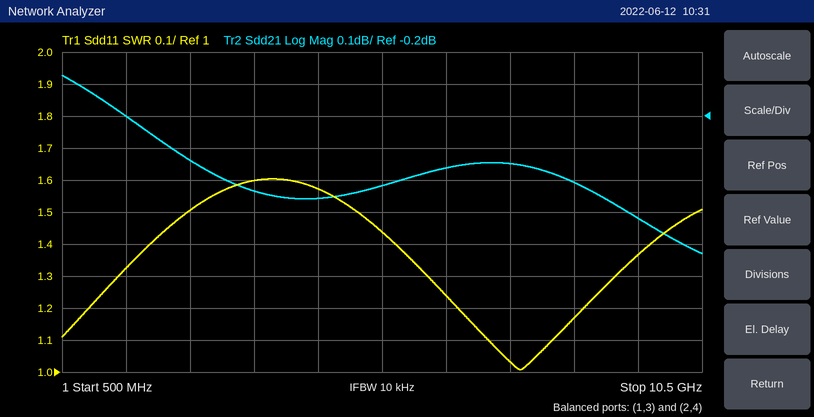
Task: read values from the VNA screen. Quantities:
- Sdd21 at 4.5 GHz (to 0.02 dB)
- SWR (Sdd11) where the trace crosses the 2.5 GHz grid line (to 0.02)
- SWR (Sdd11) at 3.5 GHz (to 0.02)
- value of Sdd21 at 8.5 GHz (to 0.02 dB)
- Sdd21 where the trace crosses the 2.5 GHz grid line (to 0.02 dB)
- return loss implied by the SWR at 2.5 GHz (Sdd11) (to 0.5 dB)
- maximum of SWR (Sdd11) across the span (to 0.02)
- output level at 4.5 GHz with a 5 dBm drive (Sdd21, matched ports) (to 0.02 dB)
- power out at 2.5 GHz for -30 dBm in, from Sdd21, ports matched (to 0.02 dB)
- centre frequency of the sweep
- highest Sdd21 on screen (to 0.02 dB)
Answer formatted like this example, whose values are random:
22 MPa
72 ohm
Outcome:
-0.46 dB
1.50
1.60
-0.40 dB
-0.34 dB
14.0 dB
1.60
4.54 dBm
-30.34 dBm
5.5 GHz
-0.08 dB
